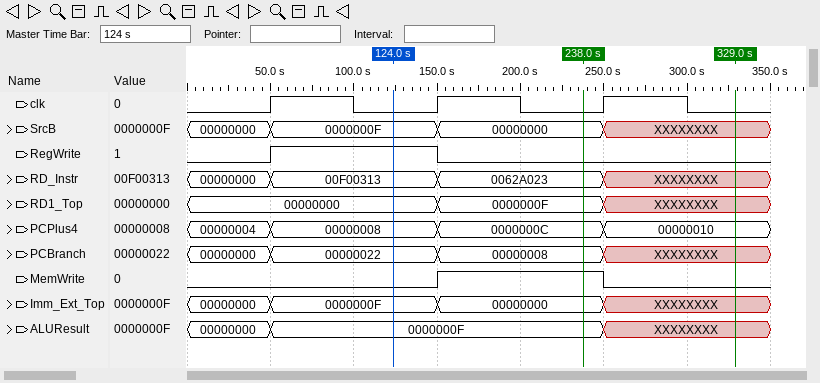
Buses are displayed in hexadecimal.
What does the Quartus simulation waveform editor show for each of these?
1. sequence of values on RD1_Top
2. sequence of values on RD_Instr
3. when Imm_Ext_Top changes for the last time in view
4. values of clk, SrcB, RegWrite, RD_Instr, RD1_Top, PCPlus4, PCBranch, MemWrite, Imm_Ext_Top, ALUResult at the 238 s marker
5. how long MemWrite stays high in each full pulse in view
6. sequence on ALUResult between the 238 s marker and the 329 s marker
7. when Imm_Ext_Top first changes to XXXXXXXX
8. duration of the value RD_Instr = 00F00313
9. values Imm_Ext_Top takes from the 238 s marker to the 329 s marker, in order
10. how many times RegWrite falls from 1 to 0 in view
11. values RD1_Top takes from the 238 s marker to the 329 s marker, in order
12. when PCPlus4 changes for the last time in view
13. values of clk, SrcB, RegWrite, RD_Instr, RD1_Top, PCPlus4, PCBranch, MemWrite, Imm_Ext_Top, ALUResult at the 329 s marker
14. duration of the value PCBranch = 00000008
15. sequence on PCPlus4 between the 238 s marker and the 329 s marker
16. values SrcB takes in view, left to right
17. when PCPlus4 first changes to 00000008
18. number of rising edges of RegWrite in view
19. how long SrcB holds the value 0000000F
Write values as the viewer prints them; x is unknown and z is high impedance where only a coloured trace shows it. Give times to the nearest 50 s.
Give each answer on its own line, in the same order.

00000000, 0000000F, XXXXXXXX
00000000, 00F00313, 0062A023, XXXXXXXX
250 s
clk=0, SrcB=00000000, RegWrite=0, RD_Instr=0062A023, RD1_Top=0000000F, PCPlus4=0000000C, PCBranch=00000008, MemWrite=1, Imm_Ext_Top=00000000, ALUResult=0000000F
100 s
0000000F, XXXXXXXX
250 s
100 s
00000000, XXXXXXXX
1
0000000F, XXXXXXXX
250 s
clk=0, SrcB=XXXXXXXX, RegWrite=0, RD_Instr=XXXXXXXX, RD1_Top=XXXXXXXX, PCPlus4=00000010, PCBranch=XXXXXXXX, MemWrite=0, Imm_Ext_Top=XXXXXXXX, ALUResult=XXXXXXXX
100 s
0000000C, 00000010
00000000, 0000000F, 00000000, XXXXXXXX
50 s
1
100 s
